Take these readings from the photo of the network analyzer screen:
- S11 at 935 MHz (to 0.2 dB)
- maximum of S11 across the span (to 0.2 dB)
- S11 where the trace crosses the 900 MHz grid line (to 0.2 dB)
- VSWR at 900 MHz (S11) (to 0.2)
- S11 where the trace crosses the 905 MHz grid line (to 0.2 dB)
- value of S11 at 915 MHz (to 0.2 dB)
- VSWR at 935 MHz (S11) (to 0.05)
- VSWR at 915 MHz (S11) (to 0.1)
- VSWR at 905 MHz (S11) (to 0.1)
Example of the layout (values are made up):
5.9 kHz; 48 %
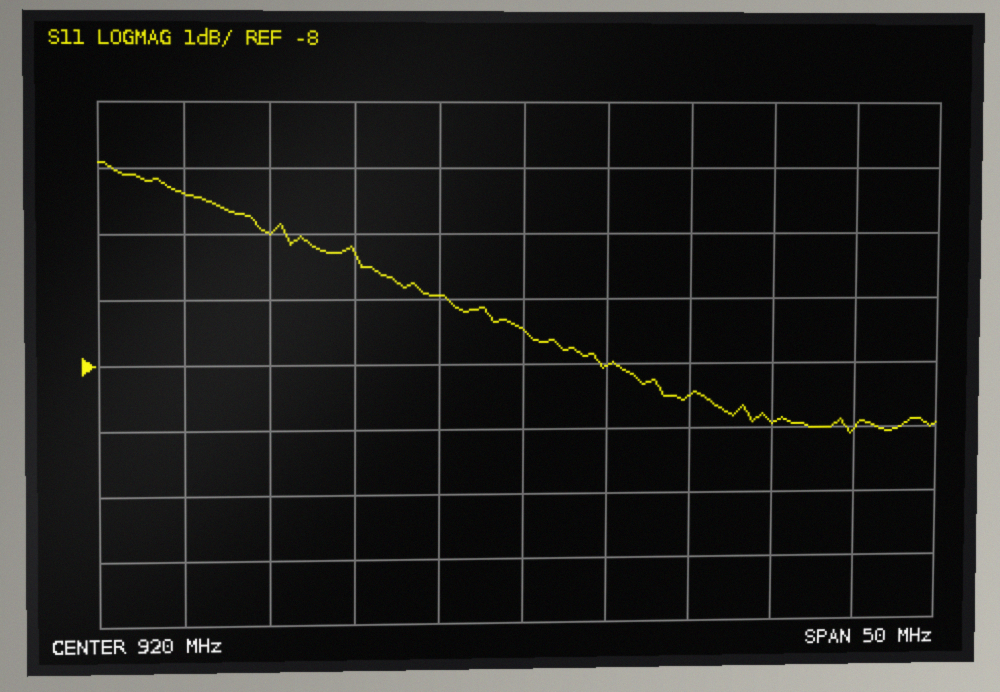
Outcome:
-9.0 dB; -5.0 dB; -5.4 dB; 3.4; -6.0 dB; -7.0 dB; 2.10; 2.6; 3.0
